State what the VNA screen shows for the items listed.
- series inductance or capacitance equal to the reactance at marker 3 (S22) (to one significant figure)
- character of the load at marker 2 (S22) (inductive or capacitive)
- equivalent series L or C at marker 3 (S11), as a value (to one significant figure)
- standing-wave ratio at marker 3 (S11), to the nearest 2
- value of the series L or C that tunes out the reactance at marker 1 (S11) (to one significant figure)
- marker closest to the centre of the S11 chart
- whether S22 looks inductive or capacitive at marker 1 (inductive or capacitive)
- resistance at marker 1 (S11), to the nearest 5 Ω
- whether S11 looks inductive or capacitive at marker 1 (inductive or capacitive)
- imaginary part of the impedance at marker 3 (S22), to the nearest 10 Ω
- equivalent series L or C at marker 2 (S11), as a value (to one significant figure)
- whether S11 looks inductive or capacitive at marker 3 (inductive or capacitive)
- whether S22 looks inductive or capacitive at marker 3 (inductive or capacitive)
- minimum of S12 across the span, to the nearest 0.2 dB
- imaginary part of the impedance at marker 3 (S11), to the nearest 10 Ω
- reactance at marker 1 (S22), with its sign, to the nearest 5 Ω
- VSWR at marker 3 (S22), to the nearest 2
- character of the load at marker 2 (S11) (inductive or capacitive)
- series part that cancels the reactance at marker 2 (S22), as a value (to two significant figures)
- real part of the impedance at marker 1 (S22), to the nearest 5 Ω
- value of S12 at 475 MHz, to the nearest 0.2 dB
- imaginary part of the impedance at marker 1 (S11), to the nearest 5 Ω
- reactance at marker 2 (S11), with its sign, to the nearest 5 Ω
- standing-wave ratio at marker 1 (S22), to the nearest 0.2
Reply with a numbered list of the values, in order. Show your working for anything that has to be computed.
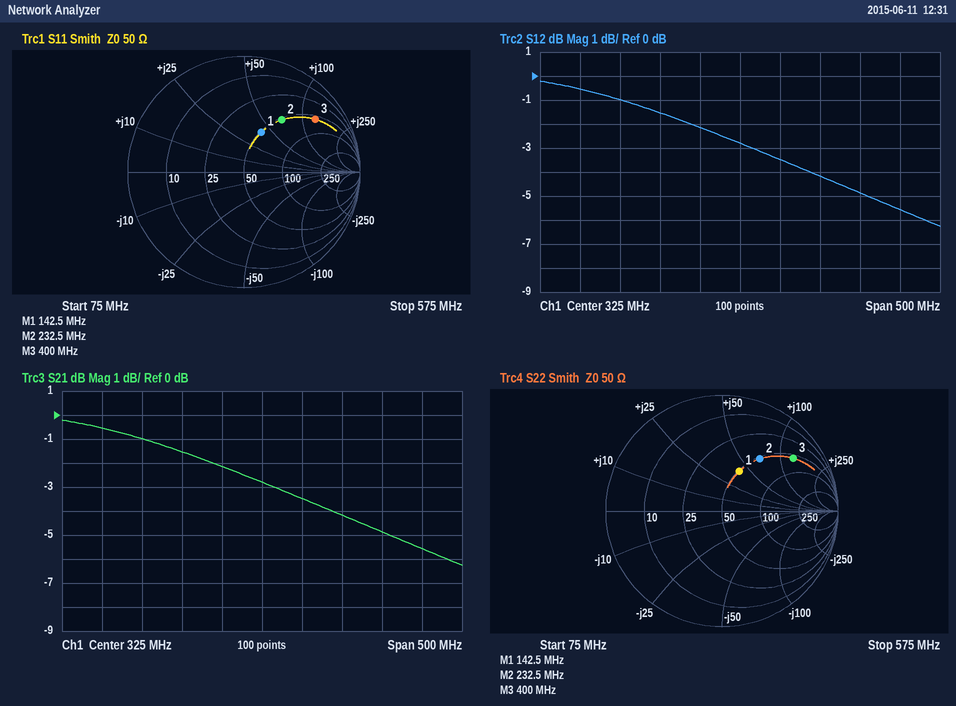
1. L = 130 Ω/(2π × 400 MHz) ≈ 51.7 nH, so 50 nH to one significant figure
2. inductive
3. L = 130 Ω/(2π × 400 MHz) ≈ 51.7 nH, so 50 nH to one significant figure
4. 8
5. C = 1/(2π × 142.5 MHz × 40 Ω) ≈ 27.9 pF, so 30 pF to one significant figure
6. marker 1
7. inductive
8. 50 Ω
9. inductive
10. +130 Ω
11. L = 70 Ω/(2π × 232.5 MHz) ≈ 47.9 nH, so 50 nH to one significant figure
12. inductive
13. inductive
14. -6.2 dB
15. +130 Ω
16. +40 Ω
17. 8
18. inductive
19. C = 1/(2π × 232.5 MHz × 70 Ω) ≈ 10 pF
20. 50 Ω
21. -4.8 dB
22. +40 Ω
23. +70 Ω
24. 2.2
